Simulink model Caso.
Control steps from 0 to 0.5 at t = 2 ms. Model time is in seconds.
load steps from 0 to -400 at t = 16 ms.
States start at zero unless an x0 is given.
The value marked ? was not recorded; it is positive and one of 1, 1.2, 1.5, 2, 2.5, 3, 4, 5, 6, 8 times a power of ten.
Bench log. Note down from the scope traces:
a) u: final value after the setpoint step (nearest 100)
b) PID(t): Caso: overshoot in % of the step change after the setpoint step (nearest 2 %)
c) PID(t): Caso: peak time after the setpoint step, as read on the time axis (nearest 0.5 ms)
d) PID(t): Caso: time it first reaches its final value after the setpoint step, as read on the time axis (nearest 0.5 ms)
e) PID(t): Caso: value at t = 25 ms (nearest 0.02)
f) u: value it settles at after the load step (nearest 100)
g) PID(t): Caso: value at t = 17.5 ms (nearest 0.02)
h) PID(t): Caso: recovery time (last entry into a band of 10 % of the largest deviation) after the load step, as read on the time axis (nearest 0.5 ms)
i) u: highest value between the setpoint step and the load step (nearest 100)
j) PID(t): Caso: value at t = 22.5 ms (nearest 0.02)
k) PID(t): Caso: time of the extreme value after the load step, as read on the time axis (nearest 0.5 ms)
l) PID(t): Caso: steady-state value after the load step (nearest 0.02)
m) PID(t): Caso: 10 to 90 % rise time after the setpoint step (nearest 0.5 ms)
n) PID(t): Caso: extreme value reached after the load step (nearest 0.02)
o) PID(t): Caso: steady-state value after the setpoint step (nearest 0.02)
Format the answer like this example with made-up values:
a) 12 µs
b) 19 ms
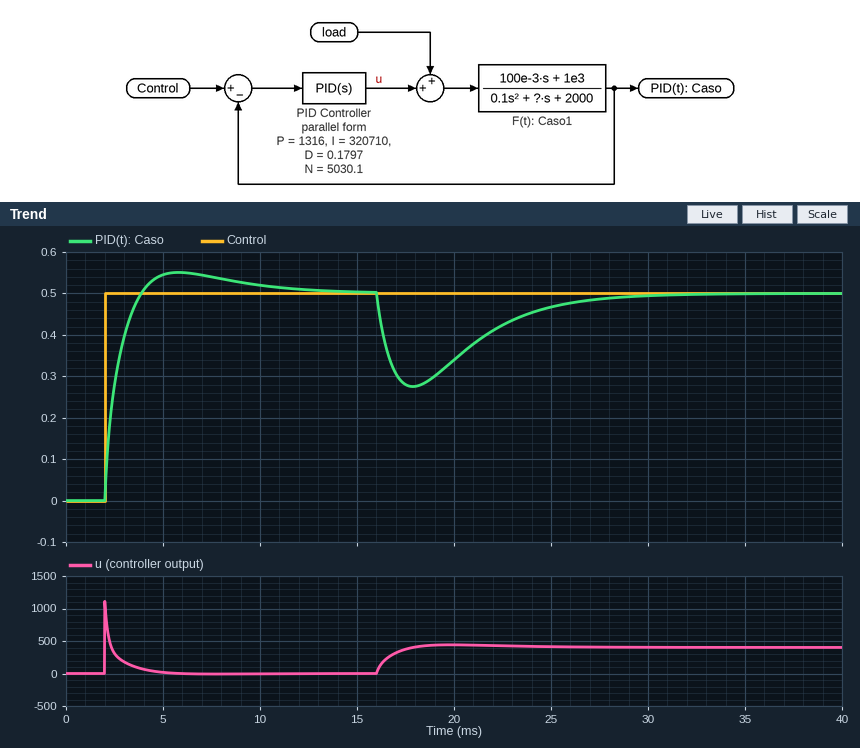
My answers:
a) 0
b) 10 %
c) 6.0 ms
d) 4.0 ms
e) 0.46
f) 400
g) 0.28
h) 26.0 ms
i) 1100
j) 0.42
k) 18.0 ms
l) 0.50
m) 1.5 ms
n) 0.28
o) 0.50
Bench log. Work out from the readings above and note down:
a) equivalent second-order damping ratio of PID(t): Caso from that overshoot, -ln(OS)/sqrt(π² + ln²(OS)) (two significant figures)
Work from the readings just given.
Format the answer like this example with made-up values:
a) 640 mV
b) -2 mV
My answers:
a) 0.59
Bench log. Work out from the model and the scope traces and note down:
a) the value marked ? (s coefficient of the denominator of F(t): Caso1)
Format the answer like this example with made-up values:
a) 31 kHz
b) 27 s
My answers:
a) 1000
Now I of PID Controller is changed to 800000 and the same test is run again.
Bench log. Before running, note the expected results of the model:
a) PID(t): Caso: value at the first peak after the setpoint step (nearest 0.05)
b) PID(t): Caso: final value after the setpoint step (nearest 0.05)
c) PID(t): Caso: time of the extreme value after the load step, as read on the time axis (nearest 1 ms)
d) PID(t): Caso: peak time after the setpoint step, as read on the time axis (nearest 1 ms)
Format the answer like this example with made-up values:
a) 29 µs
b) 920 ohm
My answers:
a) 0.60
b) 0.50
c) 17 ms
d) 5 ms
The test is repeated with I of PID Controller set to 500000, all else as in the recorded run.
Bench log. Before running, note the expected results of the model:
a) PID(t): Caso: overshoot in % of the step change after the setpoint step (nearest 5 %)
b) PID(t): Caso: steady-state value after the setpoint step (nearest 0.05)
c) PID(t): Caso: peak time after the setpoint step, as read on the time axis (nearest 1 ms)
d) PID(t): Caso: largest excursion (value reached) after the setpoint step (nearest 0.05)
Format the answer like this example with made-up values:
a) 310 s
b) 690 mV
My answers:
a) 15 %
b) 0.50
c) 5 ms
d) 0.55
